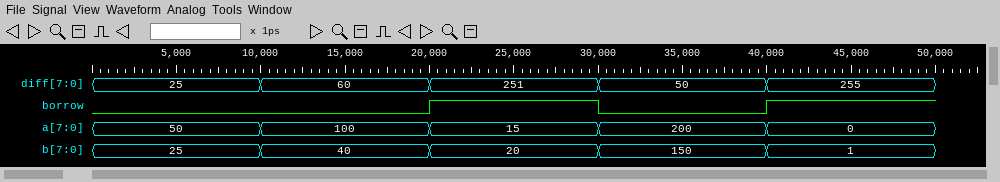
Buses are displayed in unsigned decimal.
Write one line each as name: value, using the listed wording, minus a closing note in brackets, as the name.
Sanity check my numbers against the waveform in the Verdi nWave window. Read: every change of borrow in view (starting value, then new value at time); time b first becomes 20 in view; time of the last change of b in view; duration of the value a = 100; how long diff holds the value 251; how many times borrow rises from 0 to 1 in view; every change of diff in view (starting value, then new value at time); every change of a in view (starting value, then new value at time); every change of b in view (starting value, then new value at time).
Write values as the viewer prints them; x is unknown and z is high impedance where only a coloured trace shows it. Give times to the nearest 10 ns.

every change of borrow in view: 0, 1 at 20 ns, 0 at 30 ns, 1 at 40 ns
time b first becomes 20 in view: 20 ns
time of the last change of b in view: 40 ns
duration of the value a = 100: 10 ns
how long diff holds the value 251: 10 ns
how many times borrow rises from 0 to 1 in view: 2
every change of diff in view: 25, 60 at 10 ns, 251 at 20 ns, 50 at 30 ns, 255 at 40 ns
every change of a in view: 50, 100 at 10 ns, 15 at 20 ns, 200 at 30 ns, 0 at 40 ns
every change of b in view: 25, 40 at 10 ns, 20 at 20 ns, 150 at 30 ns, 1 at 40 ns
